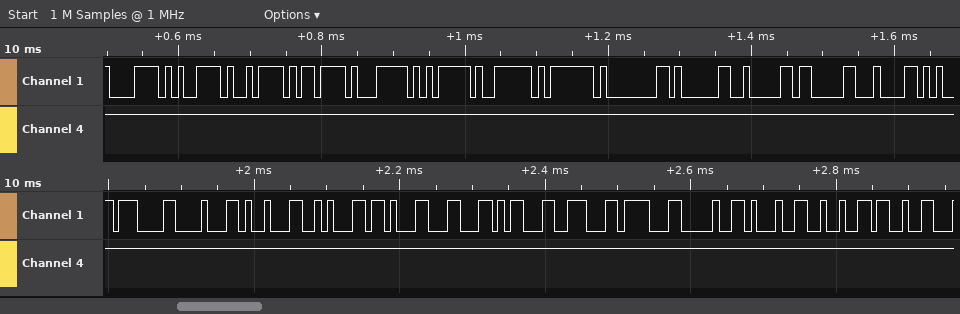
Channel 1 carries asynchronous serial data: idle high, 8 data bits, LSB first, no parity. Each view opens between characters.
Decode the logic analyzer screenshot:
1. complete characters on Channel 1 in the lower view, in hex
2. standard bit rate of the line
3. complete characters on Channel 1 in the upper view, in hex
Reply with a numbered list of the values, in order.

1. 87, 88, 89, 8A, 8B, 8C, 8D, 8E, 8F, 90, 91, 92, 93
2. 115200 baud
3. 78, 79, 7A, 7B, 7C, 7D, 7E, 7F, 80, 81, 82, 83, 84
